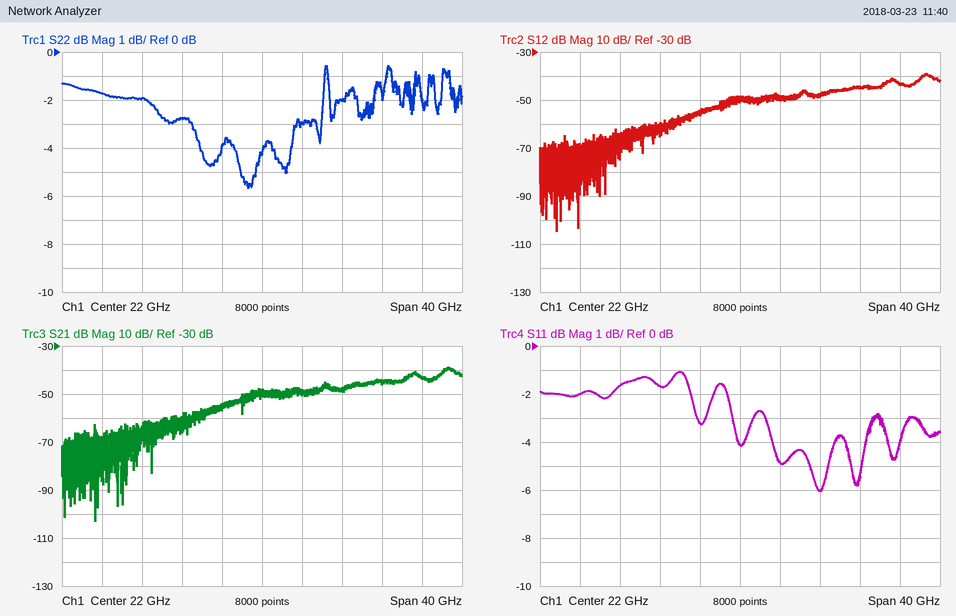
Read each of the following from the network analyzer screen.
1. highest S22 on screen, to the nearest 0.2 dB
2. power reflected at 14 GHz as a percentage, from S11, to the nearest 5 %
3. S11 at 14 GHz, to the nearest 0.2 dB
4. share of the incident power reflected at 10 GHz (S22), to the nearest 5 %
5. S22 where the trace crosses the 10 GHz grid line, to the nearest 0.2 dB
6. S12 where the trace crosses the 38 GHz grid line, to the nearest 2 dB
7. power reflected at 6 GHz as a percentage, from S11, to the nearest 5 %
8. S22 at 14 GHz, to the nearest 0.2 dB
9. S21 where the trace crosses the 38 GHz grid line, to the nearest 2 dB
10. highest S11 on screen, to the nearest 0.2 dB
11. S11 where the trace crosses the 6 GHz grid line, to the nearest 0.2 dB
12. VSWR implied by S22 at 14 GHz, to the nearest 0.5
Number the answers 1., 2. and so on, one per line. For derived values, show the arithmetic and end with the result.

1. -0.6 dB
2. 10^(-1.6/10) ≈ 69.2 %, so 70 % to the nearest 5 %
3. -1.6 dB
4. 10^(-2/10) ≈ 63.1 %, so 65 % to the nearest 5 %
5. -2.0 dB
6. -44 dB
7. 10^(-2/10) ≈ 63.1 %, so 65 % to the nearest 5 %
8. -2.8 dB
9. -44 dB
10. -1.0 dB
11. -2.0 dB
12. |Γ| = 10^(-2.8/20) = 0.7244; VSWR = (1 + 0.7244)/(1 − 0.7244) ≈ 6.26, so 6.5 to the nearest 0.5
